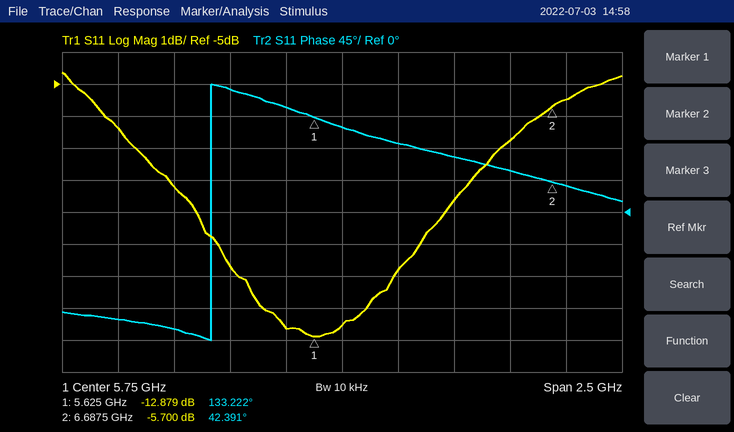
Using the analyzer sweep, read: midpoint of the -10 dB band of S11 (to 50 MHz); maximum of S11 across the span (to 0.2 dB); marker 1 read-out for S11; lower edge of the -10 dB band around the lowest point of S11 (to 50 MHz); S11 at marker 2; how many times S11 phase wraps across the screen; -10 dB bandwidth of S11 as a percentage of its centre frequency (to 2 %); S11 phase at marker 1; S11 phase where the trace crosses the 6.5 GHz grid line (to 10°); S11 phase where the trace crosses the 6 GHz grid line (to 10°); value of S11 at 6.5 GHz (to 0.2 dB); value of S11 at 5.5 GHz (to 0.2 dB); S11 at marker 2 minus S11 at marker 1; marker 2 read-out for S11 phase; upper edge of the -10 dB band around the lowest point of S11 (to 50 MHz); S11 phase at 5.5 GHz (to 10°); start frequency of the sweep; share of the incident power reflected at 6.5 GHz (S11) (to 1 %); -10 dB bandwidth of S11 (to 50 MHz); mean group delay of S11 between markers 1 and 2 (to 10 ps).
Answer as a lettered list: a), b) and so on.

a) 5.65 GHz
b) -4.6 dB
c) -12.879 dB
d) 5.20 GHz
e) -5.700 dB
f) 1
g) 16 %
h) 133.222°
i) 60°
j) 100°
k) -6.8 dB
l) -12.6 dB
m) 7.179 dB
n) 42.391°
o) 6.10 GHz
p) 150°
q) 4.5 GHz
r) 21 %
s) 900 MHz
t) 240 ps
